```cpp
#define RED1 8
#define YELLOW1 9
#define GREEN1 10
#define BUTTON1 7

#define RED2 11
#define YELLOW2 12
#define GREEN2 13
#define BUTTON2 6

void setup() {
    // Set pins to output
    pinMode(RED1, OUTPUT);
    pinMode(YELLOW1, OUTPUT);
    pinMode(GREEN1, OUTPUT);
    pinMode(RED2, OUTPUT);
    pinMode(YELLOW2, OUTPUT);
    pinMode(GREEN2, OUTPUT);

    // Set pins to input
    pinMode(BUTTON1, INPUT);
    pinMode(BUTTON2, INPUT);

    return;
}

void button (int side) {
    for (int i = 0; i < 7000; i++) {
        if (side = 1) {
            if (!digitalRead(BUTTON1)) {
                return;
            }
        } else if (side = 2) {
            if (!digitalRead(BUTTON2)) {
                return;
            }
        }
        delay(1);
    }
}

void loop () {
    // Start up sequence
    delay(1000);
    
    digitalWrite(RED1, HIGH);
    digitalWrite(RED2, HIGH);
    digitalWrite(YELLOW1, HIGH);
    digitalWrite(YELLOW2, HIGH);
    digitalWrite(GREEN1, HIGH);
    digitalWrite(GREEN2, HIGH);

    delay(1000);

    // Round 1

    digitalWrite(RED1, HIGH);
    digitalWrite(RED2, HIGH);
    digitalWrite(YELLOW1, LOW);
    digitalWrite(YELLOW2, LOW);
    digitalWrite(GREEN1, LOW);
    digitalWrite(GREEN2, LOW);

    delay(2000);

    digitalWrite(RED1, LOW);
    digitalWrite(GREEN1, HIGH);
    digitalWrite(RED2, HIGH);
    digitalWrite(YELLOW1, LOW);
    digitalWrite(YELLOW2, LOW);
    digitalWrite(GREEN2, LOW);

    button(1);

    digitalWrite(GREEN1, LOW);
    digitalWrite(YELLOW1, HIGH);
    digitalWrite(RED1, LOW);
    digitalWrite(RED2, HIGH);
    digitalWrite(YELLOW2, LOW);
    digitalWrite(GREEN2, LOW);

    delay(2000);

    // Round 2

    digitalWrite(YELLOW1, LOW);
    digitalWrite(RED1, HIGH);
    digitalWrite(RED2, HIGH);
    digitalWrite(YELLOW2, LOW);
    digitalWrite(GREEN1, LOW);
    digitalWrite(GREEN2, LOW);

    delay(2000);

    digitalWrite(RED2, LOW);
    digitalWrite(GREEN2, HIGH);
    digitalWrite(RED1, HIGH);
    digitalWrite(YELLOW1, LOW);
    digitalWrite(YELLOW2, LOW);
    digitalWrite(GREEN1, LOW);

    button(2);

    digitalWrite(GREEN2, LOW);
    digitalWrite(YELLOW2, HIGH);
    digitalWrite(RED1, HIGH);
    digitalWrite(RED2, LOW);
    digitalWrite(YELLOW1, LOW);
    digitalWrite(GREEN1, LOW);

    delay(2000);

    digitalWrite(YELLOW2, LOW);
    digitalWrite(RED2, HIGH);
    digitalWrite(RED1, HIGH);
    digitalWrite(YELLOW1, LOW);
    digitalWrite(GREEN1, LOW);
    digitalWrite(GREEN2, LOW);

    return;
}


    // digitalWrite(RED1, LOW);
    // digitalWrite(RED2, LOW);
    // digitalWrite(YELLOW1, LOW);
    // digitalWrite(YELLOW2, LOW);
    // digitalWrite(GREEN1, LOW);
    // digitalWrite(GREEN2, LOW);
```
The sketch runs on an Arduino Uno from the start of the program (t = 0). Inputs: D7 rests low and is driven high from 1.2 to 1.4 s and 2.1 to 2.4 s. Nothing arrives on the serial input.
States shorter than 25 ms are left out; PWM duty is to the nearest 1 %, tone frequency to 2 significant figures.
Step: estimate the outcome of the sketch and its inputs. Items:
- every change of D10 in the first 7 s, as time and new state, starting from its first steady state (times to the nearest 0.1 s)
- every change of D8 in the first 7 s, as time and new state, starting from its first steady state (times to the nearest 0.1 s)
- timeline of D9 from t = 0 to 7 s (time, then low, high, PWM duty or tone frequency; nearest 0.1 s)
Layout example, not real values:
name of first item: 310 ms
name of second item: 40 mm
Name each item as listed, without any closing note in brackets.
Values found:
every change of D10 in the first 7 s, as time and new state, starting from its first steady state: 0 s low; 1 s high; 2 s low
every change of D8 in the first 7 s, as time and new state, starting from its first steady state: 0 s low; 1 s high; 4 s low; 6 s high
timeline of D9 from t = 0 to 7 s: 0 s low; 1 s high; 2 s low; 4 s high; 6 s low
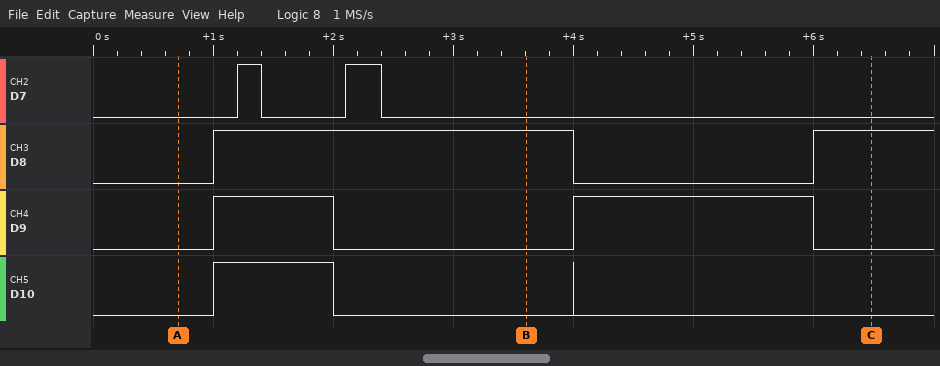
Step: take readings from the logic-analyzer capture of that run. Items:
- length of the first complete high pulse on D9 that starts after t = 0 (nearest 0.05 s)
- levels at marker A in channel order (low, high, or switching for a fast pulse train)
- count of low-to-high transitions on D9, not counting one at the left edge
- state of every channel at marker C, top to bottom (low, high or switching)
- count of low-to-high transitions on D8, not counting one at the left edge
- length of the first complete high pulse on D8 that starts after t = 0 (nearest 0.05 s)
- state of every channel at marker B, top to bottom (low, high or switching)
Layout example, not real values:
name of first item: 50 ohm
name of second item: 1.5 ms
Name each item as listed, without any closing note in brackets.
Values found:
length of the first complete high pulse on D9 that starts after t = 0: 1.00 s
levels at marker A in channel order: D7 low, D8 low, D9 low, D10 low
count of low-to-high transitions on D9, not counting one at the left edge: 2
state of every channel at marker C, top to bottom: D7 low, D8 high, D9 low, D10 low
count of low-to-high transitions on D8, not counting one at the left edge: 2
length of the first complete high pulse on D8 that starts after t = 0: 3.00 s
state of every channel at marker B, top to bottom: D7 low, D8 high, D9 low, D10 low
